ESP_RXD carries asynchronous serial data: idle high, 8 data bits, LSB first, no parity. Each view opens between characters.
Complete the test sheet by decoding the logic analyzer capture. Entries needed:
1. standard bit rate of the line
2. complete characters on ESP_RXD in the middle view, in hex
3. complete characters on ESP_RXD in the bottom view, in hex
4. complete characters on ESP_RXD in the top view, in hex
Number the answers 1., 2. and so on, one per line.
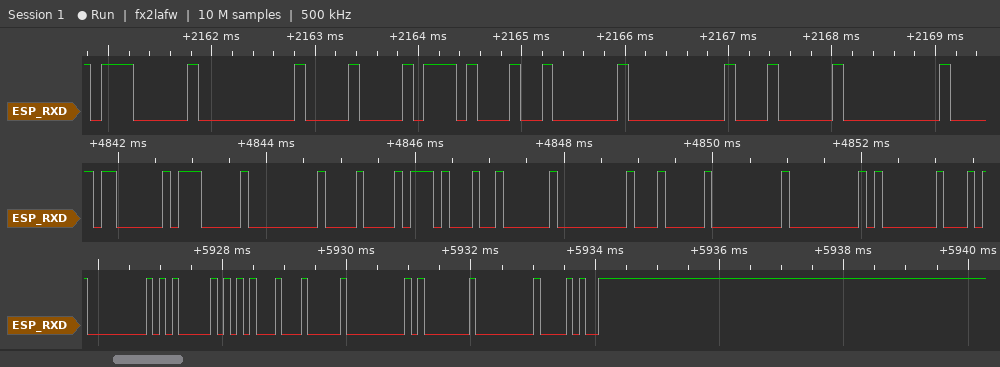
1. 9600 baud
2. 03, 07, 00, 08, 17, 02, 00, 04, 00, 00, 01
3. 00, 05, 15, 04, 00, 01, 00, 28
4. 07, 00, 08, 17, 02, 00, 04, 00
